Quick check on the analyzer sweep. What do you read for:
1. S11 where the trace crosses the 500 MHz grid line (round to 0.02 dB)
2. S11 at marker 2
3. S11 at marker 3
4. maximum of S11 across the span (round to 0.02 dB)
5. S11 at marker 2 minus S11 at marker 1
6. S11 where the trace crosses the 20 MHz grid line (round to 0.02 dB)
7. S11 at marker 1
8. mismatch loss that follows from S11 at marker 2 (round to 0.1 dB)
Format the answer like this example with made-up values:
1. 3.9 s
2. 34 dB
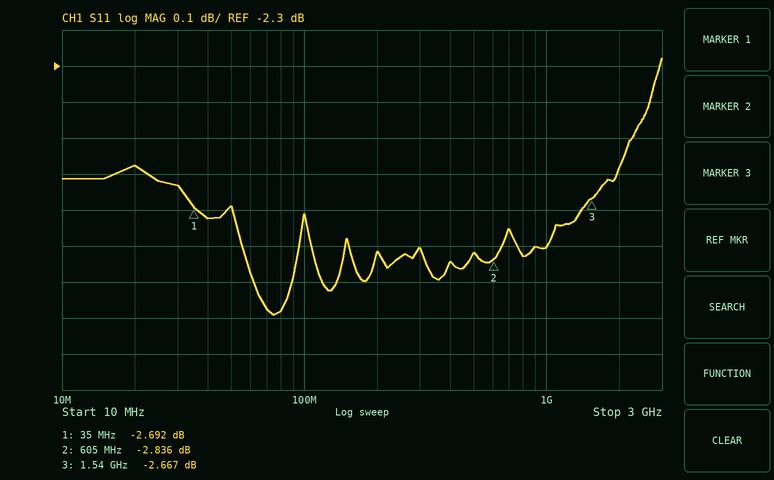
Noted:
1. -2.82 dB
2. -2.836 dB
3. -2.667 dB
4. -2.28 dB
5. -0.144 dB
6. -2.58 dB
7. -2.692 dB
8. 3.2 dB
